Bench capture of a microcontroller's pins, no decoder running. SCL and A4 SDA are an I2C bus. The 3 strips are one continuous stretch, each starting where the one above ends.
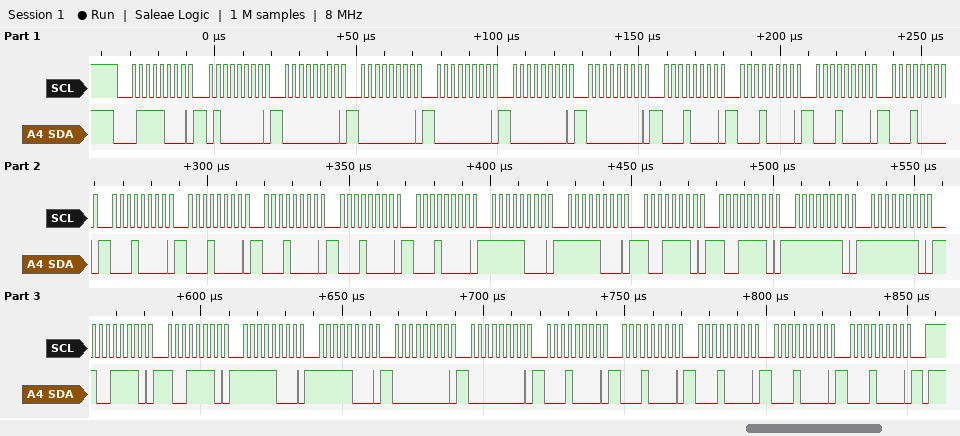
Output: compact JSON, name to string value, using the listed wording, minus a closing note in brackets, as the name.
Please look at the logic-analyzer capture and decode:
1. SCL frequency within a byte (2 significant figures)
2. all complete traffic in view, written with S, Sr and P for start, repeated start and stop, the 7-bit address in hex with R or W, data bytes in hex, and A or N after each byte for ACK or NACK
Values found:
{"SCL frequency within a byte": "400 kHz", "all complete traffic in view, written with S, Sr and P for start, repeated start and stop, the 7-bit address in hex with R or W, data bytes in hex, and A or N after each byte for ACK or NACK": "S 3CW A 40 A 00 A 00 A 00 A 00 A 00 A 10 A 10 A 10 A 10 A 10 A 10 A 10 A 10 A 10 A F8 A F8 A 9E A 9E A FE A FE A 9E A 9E A F8 A F8 A 00 A 00 A 10 A 10 A 10 A 10 A 10 A P"}
